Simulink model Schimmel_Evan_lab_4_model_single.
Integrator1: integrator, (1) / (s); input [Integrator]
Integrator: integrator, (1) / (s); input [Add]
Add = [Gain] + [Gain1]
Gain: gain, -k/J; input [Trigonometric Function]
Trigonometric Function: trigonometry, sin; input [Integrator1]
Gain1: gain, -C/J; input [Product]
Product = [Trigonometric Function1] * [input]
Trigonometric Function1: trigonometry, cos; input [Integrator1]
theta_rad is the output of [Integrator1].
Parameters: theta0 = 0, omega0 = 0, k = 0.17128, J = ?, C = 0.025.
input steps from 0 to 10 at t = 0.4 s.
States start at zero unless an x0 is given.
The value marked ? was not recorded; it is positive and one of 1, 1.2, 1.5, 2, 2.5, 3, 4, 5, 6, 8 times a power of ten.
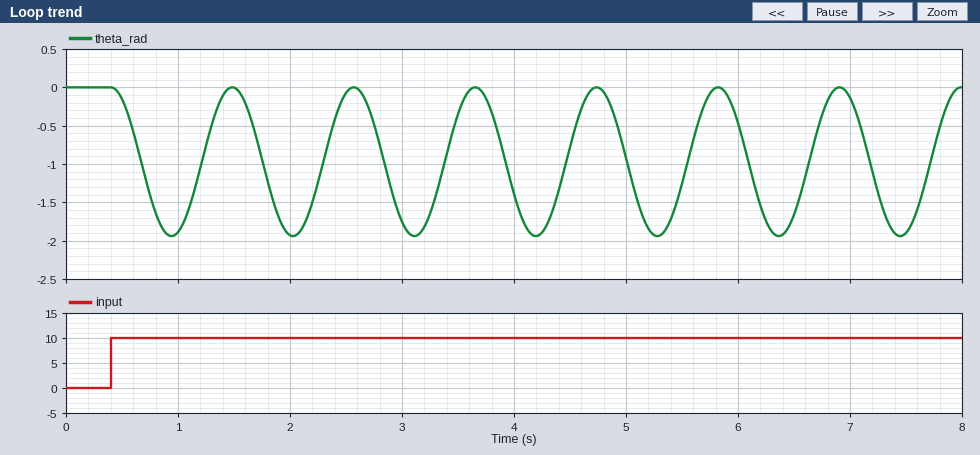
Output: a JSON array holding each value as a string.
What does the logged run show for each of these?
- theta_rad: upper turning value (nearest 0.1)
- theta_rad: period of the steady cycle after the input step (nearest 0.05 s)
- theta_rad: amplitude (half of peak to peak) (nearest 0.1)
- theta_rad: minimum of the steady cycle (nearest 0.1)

["0.0", "1.10 s", "1.0", "-1.9"]
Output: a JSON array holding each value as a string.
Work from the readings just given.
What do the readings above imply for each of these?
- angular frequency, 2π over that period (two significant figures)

["5.7 rad/s"]
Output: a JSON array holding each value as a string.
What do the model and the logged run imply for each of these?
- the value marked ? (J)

["0.008"]
